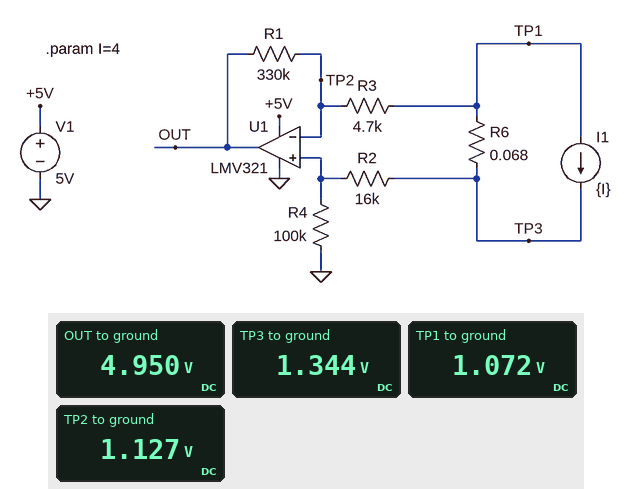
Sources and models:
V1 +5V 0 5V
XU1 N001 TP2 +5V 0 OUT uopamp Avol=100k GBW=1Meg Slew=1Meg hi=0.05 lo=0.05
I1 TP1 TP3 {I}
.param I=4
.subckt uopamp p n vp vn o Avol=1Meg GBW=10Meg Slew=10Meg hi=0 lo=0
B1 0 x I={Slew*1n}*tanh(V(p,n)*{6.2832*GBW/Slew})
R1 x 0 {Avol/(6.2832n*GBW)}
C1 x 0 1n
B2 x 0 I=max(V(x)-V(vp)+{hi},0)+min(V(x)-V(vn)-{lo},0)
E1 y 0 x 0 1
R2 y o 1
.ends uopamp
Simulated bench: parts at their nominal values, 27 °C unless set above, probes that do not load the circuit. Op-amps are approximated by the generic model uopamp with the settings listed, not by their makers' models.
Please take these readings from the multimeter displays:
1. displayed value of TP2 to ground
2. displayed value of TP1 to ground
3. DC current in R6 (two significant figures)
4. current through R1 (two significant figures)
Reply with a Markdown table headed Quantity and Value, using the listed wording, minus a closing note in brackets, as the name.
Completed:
| Quantity | Value |
|---|---|
| displayed value of TP2 to ground | 1.127 V |
| displayed value of TP1 to ground | 1.072 V |
| DC current in R6 | 4.0 A |
| current through R1 | 12 µA |
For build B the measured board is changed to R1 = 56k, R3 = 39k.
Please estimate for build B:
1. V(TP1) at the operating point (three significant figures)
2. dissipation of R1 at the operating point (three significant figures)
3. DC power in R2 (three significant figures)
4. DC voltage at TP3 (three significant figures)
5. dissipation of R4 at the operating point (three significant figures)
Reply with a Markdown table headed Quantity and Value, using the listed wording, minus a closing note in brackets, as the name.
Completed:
| Quantity | Value |
|---|---|
| V(TP1) at the operating point | 302 mV |
| dissipation of R1 at the operating point | 1.37 µW |
| DC power in R2 | 391 nW |
| DC voltage at TP3 | 574 mV |
| dissipation of R4 at the operating point | 2.45 µW |
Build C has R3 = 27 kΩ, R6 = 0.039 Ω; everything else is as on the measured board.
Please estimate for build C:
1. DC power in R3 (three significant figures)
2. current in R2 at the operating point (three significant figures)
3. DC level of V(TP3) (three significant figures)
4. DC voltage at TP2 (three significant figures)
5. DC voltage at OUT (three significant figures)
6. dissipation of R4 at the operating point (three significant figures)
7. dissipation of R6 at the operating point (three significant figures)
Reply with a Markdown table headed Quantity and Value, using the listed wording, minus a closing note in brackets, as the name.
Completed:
| Quantity | Value |
|---|---|
| DC power in R3 | 355 nW |
| current in R2 at the operating point | 3.63 µA |
| DC level of V(TP3) | 421 mV |
| DC voltage at TP2 | 363 mV |
| DC voltage at OUT | 1.56 V |
| dissipation of R4 at the operating point | 1.32 µW |
| dissipation of R6 at the operating point | 624 mW |
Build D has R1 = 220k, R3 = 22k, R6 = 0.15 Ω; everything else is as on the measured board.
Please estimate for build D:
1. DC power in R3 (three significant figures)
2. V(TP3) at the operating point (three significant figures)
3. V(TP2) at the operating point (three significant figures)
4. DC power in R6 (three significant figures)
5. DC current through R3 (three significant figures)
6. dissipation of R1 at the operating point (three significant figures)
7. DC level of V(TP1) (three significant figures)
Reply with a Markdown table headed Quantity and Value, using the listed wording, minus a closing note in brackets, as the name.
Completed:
| Quantity | Value |
|---|---|
| DC power in R3 | 5.29 µW |
| V(TP3) at the operating point | 1.80 V |
| V(TP2) at the operating point | 1.54 V |
| DC power in R6 | 2.40 W |
| DC current through R3 | 15.5 µA |
| dissipation of R1 at the operating point | 52.9 µW |
| DC level of V(TP1) | 1.20 V |
